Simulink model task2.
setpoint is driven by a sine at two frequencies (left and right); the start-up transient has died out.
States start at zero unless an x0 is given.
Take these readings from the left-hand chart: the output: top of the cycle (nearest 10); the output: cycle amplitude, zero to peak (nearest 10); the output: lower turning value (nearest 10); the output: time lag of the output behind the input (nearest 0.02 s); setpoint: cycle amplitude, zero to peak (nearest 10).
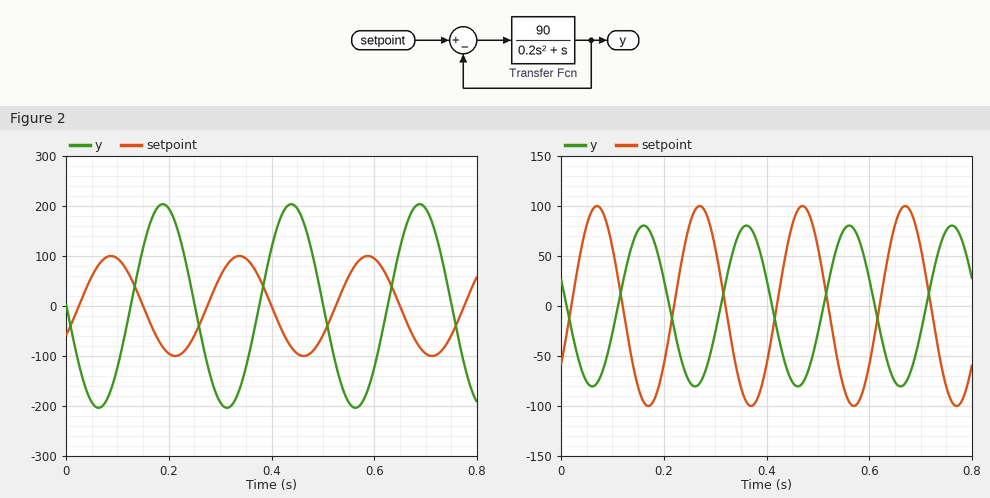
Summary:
200
200
-200
0.10 s
100
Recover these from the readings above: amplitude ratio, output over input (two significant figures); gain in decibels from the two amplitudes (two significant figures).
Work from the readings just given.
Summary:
2.0
6.0 dB
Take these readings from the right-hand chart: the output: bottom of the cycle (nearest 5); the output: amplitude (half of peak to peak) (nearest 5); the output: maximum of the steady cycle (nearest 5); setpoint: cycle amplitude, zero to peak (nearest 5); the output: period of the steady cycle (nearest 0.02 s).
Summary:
-80
80
80
100
0.20 s
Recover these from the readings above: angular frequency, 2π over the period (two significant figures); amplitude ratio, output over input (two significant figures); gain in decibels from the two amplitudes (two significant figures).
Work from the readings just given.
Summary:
31 rad/s
0.80
-1.9 dB
